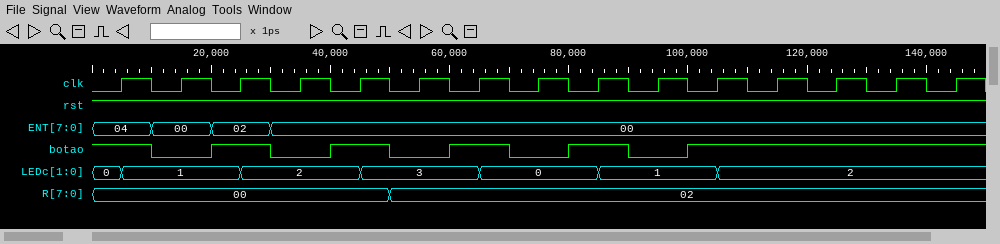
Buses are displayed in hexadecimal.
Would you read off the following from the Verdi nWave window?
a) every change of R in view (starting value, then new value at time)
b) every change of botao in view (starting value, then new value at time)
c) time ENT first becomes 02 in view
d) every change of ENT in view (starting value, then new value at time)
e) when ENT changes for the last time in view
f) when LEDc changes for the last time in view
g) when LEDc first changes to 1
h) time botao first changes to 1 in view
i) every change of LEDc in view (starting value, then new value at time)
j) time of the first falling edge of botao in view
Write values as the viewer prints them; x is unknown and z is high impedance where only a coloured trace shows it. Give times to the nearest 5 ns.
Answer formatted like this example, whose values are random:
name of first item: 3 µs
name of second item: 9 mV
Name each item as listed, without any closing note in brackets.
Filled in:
every change of R in view: 00, 02 at 50 ns
every change of botao in view: 1, 0 at 10 ns, 1 at 20 ns, 0 at 30 ns, 1 at 40 ns, 0 at 50 ns, 1 at 60 ns, 0 at 70 ns, 1 at 80 ns, 0 at 90 ns, 1 at 100 ns
time ENT first becomes 02 in view: 20 ns
every change of ENT in view: 04, 00 at 10 ns, 02 at 20 ns, 00 at 30 ns
when ENT changes for the last time in view: 30 ns
when LEDc changes for the last time in view: 105 ns
when LEDc first changes to 1: 5 ns
time botao first changes to 1 in view: 20 ns
every change of LEDc in view: 0, 1 at 5 ns, 2 at 25 ns, 3 at 45 ns, 0 at 65 ns, 1 at 85 ns, 2 at 105 ns
time of the first falling edge of botao in view: 10 ns
